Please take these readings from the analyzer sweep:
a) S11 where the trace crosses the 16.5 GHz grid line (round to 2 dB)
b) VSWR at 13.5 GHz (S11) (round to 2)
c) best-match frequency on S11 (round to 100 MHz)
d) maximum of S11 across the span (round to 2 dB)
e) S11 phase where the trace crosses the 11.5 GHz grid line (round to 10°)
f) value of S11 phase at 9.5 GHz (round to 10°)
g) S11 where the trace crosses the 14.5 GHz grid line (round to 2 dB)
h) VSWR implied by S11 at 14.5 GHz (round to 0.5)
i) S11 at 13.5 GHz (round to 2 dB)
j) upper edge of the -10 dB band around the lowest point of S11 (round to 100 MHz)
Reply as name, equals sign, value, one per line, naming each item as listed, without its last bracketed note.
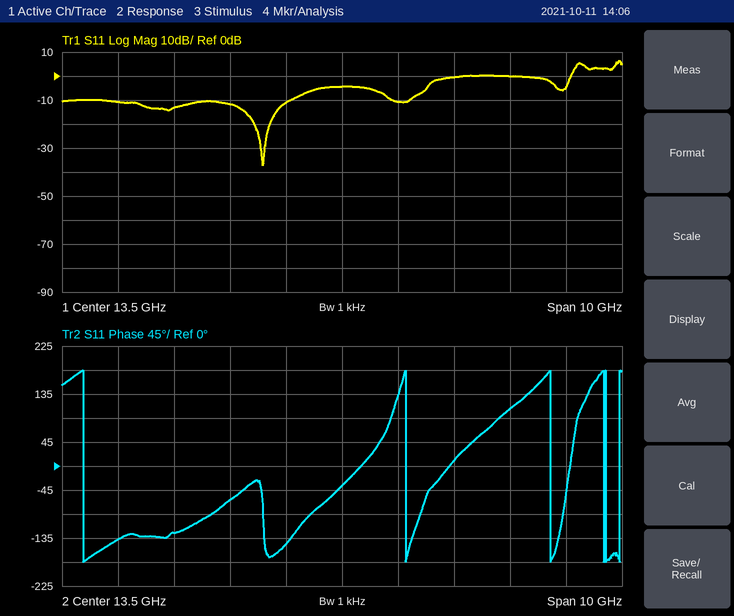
S11 where the trace crosses the 16.5 GHz grid line = 0 dB
VSWR at 13.5 GHz (S11) = 4
best-match frequency on S11 = 12.1 GHz
maximum of S11 across the span = 6 dB
S11 phase where the trace crosses the 11.5 GHz grid line = -60°
value of S11 phase at 9.5 GHz = -140°
S11 where the trace crosses the 14.5 GHz grid line = -10 dB
VSWR implied by S11 at 14.5 GHz = 2.0
S11 at 13.5 GHz = -4 dB
upper edge of the -10 dB band around the lowest point of S11 = 12.6 GHz
